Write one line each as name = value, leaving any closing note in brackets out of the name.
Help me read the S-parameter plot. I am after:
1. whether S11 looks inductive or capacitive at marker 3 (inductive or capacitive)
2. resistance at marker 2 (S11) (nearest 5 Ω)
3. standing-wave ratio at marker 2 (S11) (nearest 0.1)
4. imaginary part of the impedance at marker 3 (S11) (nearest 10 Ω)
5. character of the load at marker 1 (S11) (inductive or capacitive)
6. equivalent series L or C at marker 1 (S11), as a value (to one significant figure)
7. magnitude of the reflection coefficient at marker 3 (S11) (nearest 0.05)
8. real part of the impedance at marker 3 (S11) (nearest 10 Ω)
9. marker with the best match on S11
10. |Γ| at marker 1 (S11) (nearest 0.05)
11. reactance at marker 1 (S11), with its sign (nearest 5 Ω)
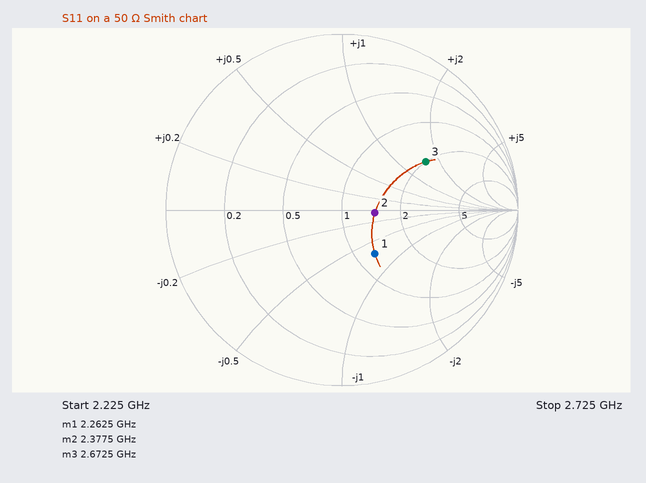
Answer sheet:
whether S11 looks inductive or capacitive at marker 3 = inductive
resistance at marker 2 (S11) = 75 Ω
standing-wave ratio at marker 2 (S11) = 1.5
imaginary part of the impedance at marker 3 (S11) = +80 Ω
character of the load at marker 1 (S11) = capacitive
equivalent series L or C at marker 1 (S11), as a value = 2 pF
magnitude of the reflection coefficient at marker 3 (S11) = 0.55
real part of the impedance at marker 3 (S11) = 100 Ω
marker with the best match on S11 = marker 2
|Γ| at marker 1 (S11) = 0.30
reactance at marker 1 (S11), with its sign = -35 Ω
